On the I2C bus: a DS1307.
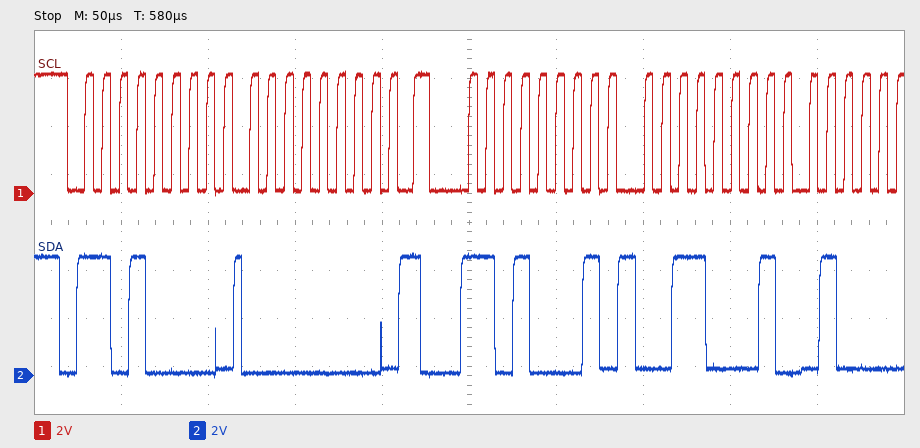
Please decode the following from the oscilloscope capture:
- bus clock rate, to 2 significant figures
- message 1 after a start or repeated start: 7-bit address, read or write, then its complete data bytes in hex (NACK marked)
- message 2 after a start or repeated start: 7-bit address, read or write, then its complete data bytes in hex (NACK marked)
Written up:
100 kHz
0x68 write: 00
0x68 read: 31
